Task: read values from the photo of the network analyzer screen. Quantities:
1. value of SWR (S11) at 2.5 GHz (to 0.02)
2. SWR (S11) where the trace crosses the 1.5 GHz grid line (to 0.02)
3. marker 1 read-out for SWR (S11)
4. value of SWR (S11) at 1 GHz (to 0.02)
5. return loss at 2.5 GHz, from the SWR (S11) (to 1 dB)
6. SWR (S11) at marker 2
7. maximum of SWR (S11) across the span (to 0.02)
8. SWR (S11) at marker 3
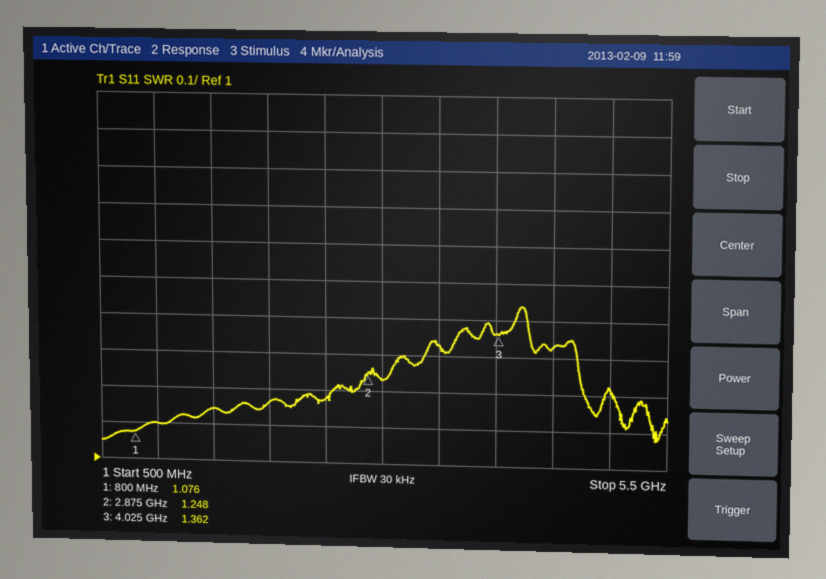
1.18
1.14
1.076
1.10
22 dB
1.248
1.44
1.362
